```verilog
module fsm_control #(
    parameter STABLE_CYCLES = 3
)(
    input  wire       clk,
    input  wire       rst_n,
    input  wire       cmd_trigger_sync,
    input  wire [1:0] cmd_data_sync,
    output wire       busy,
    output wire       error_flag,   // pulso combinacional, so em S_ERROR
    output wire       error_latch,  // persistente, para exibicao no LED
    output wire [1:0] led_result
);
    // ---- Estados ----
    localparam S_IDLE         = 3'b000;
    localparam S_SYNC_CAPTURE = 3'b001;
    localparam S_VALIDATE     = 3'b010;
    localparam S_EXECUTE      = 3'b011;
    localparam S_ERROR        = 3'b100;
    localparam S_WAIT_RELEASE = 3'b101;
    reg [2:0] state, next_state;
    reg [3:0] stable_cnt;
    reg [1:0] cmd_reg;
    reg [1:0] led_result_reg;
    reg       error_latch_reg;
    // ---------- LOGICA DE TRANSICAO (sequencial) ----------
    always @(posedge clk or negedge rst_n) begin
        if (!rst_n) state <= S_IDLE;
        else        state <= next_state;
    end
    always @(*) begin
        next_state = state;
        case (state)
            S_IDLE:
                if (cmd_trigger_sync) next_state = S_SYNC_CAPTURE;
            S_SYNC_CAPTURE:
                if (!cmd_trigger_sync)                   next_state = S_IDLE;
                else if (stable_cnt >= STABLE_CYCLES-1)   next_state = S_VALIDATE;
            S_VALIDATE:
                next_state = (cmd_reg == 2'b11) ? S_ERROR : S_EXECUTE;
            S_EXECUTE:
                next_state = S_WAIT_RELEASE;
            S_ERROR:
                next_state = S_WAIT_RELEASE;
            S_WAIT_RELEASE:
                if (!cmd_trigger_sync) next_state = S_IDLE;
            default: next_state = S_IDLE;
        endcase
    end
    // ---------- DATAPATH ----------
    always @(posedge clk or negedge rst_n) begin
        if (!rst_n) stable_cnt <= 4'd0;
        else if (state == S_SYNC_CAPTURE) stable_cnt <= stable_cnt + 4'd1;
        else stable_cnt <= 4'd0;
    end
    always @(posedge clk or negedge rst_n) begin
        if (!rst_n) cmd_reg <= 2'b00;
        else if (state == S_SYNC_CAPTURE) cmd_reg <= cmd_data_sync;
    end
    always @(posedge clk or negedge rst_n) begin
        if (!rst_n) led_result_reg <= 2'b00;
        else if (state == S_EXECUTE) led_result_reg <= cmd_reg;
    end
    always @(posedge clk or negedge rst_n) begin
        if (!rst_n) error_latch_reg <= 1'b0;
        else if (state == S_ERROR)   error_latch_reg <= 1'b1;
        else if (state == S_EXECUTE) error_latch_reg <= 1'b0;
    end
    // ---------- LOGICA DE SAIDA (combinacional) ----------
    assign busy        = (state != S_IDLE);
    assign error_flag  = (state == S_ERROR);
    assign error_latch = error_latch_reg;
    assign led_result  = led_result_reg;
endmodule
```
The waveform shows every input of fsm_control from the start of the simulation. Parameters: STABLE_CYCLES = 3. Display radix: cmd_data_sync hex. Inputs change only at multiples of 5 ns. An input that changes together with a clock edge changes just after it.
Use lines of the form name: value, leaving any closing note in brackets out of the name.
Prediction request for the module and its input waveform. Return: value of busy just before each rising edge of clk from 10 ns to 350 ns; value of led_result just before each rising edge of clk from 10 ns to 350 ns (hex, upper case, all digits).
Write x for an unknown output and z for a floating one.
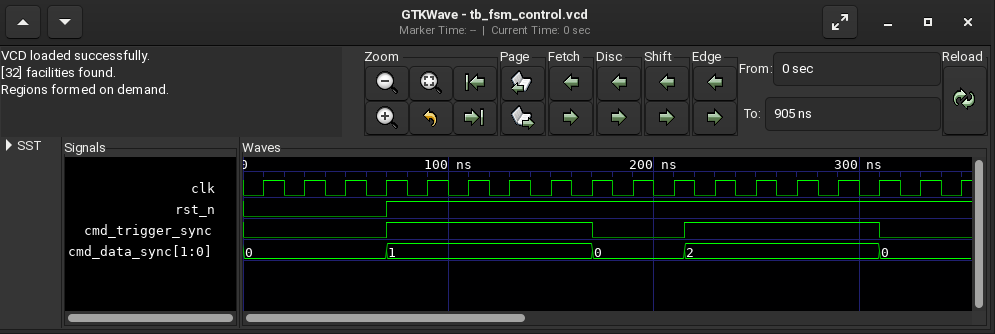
value of busy just before each rising edge of clk from 10 ns to 350 ns: 0 0 0 0 0 1 1 1 1 1 1 0 1 1 1 1 1 1
value of led_result just before each rising edge of clk from 10 ns to 350 ns: 0, 0, 0, 0, 0, 0, 0, 0, 0, 0, 1, 1, 1, 1, 1, 1, 1, 2
